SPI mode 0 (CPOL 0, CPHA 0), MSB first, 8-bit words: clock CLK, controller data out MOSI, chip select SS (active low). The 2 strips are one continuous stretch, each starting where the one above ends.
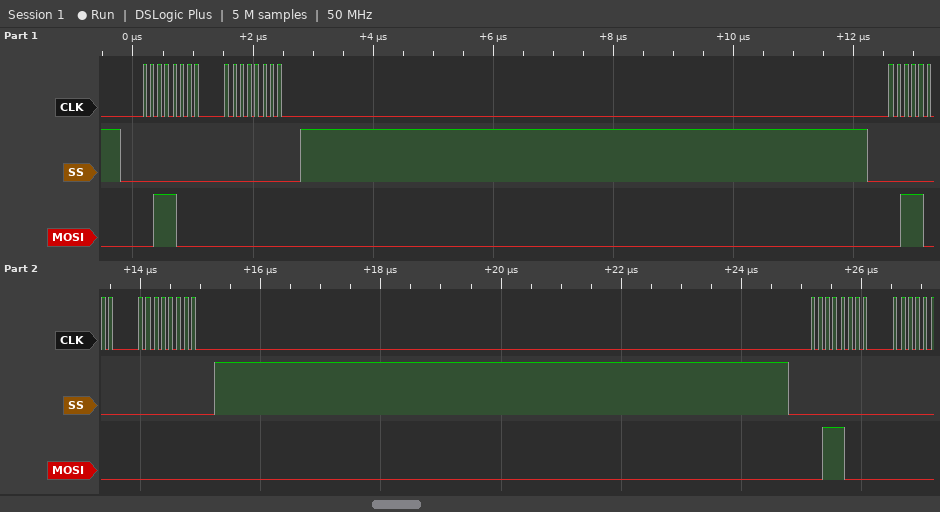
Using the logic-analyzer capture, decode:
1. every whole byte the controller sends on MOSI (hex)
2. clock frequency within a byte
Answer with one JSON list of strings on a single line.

["38 00 38 00 38", "8 MHz"]
